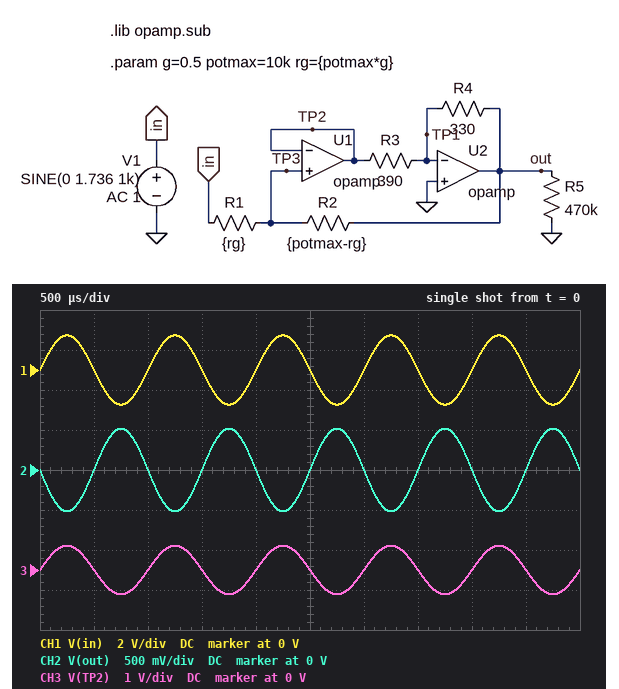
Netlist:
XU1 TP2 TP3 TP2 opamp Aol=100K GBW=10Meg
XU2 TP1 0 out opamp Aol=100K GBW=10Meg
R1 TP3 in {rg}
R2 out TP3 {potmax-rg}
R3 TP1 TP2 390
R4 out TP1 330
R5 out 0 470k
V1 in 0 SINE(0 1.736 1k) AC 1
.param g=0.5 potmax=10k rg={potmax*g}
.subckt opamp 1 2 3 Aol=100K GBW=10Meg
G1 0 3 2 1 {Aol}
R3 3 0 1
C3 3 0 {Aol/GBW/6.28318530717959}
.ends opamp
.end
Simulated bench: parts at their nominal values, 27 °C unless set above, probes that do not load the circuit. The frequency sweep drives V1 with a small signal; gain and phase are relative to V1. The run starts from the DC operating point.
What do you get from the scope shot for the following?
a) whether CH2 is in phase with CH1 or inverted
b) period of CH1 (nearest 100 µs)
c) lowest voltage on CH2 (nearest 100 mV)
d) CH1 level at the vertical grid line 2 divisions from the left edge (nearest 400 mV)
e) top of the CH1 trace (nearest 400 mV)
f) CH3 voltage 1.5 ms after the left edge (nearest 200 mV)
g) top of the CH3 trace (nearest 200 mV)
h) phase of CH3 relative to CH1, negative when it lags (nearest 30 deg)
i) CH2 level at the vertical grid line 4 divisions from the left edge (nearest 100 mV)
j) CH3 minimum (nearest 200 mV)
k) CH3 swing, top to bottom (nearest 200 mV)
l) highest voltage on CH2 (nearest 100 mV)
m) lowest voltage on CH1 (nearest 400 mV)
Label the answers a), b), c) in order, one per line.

a) inverted
b) 1.0 ms
c) -500 mV
d) 0 V
e) 1.6 V
f) 0 V
g) 600 mV
h) 0 deg
i) 0 V
j) -600 mV
k) 1.2 V
l) 500 mV
m) -1.6 V
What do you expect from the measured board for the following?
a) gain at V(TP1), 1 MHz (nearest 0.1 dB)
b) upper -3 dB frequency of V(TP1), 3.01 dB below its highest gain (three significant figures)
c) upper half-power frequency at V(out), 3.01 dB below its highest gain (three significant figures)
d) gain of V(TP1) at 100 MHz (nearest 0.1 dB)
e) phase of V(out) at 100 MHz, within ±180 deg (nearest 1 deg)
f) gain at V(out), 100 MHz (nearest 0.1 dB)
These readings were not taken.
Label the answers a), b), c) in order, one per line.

a) -30.6 dB
b) 19.4 MHz
c) 6.78 MHz
d) -32.8 dB
e) 9 deg
f) -52.8 dB
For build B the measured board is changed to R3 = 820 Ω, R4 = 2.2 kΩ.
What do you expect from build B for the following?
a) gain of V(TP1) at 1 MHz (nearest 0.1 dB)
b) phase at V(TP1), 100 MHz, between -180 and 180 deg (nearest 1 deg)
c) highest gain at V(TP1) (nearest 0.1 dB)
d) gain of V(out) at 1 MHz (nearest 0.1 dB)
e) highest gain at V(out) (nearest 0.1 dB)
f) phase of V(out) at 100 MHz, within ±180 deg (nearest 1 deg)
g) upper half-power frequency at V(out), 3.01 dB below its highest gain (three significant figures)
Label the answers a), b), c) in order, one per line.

a) -24.9 dB
b) -83 deg
c) -10.9 dB
d) -4.9 dB
e) -4.8 dB
f) 7 deg
g) 6.97 MHz
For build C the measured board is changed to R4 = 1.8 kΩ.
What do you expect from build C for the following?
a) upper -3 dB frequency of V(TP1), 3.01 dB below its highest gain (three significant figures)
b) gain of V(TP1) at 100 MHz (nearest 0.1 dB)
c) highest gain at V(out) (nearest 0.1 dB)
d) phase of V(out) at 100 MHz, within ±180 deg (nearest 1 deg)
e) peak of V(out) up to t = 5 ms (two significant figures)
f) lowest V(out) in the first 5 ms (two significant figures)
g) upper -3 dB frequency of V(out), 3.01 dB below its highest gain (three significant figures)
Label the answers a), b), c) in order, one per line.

a) 15.6 MHz
b) -27.7 dB
c) -3.1 dB
d) 7 deg
e) 1.2 V
f) -1.2 V
g) 7.02 MHz
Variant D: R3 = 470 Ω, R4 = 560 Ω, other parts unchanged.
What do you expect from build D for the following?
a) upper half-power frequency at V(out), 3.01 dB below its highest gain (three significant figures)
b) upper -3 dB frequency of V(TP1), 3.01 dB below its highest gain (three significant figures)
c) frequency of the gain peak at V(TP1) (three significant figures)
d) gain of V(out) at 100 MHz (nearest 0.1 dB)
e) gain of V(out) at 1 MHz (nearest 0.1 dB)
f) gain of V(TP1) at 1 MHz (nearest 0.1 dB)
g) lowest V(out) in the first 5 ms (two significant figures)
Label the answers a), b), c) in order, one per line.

a) 6.84 MHz
b) 18.5 MHz
c) 8.53 MHz
d) -51.3 dB
e) -8.6 dB
f) -28.6 dB
g) -650 mV
